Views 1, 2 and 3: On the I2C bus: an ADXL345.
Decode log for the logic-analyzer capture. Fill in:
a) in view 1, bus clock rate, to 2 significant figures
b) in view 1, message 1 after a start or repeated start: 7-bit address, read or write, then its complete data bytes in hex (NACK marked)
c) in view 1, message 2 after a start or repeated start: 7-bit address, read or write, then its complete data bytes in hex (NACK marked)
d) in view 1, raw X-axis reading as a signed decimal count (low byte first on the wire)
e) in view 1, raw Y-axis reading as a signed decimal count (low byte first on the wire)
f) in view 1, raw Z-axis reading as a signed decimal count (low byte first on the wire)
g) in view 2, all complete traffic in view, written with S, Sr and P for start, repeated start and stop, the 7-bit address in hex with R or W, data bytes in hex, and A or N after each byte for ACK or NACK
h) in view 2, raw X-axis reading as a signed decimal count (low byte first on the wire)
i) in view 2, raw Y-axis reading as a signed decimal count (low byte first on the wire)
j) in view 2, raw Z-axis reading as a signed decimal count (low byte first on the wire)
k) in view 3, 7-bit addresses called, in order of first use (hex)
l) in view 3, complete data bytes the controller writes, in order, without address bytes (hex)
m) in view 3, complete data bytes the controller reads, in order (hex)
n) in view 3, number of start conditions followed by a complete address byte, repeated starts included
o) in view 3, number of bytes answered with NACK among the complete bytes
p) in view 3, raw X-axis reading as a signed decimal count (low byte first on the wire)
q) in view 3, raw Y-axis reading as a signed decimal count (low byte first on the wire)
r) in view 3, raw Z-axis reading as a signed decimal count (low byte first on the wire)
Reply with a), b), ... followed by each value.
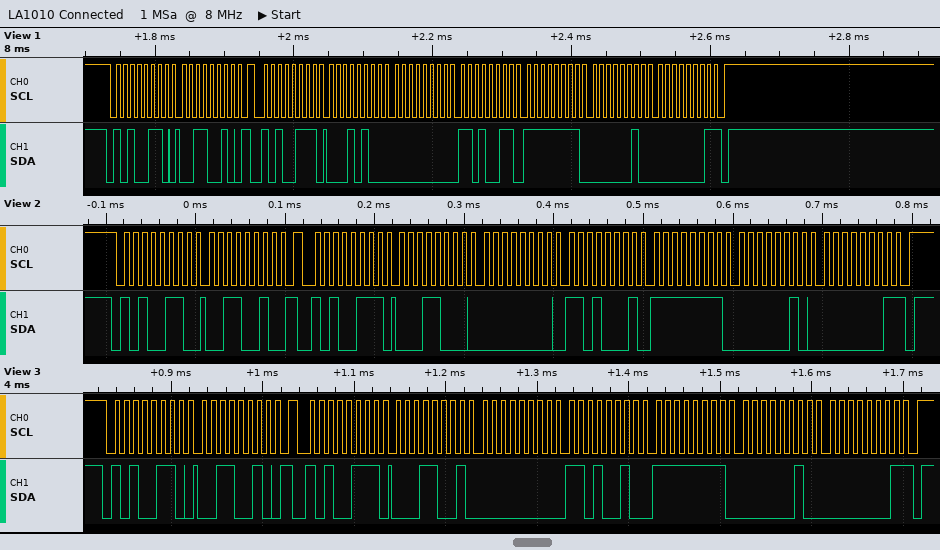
a) 100 kHz
b) 0x53 write: 32
c) 0x53 read: 14 00 D3 FF 02 01 NACK
d) 20
e) -45
f) 258
g) S 53W A 32 A Sr 53R A 18 A 00 A D1 A FF A 02 A 01 N P
h) 24
i) -47
j) 258
k) 0x53
l) 32
m) 19 00 D2 FF 02 01
n) 2
o) 1
p) 25
q) -46
r) 258
